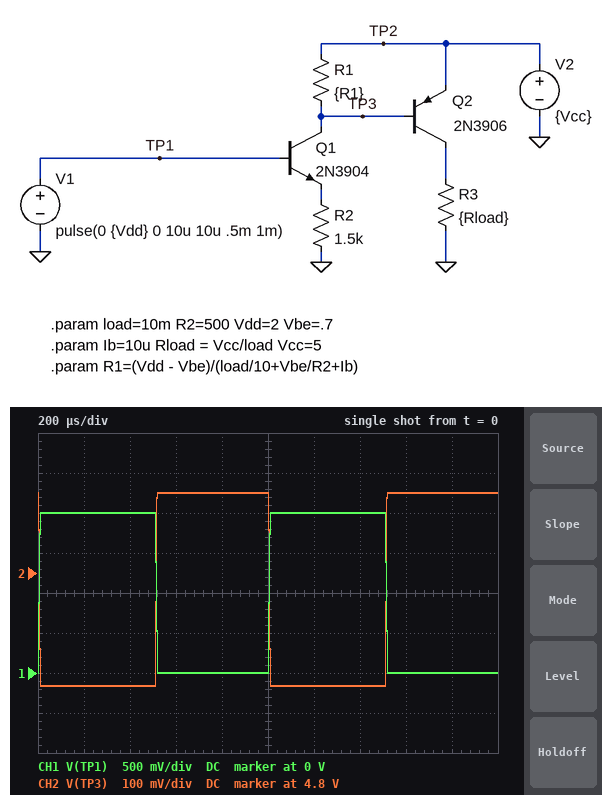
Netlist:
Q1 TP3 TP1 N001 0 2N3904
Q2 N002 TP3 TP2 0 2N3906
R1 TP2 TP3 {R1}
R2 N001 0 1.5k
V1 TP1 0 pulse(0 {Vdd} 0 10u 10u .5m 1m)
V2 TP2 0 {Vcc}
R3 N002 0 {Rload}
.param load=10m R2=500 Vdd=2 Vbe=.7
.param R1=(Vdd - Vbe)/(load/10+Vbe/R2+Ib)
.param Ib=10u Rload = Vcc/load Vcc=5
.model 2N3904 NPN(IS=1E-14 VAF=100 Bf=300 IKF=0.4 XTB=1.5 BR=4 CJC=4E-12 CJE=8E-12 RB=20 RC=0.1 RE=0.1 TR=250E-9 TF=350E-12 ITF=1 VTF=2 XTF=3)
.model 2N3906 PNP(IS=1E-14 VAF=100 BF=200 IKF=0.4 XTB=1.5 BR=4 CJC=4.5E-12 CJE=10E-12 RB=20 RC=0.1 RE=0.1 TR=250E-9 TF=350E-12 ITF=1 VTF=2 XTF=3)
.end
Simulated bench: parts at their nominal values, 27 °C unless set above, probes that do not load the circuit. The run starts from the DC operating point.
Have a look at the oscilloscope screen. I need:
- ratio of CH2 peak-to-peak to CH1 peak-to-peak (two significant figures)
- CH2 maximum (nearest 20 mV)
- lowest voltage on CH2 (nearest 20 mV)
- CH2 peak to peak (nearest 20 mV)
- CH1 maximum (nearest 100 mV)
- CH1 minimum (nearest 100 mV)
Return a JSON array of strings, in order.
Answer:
["0.24", "5.00 V", "4.52 V", "480 mV", "2.0 V", "0 V"]
